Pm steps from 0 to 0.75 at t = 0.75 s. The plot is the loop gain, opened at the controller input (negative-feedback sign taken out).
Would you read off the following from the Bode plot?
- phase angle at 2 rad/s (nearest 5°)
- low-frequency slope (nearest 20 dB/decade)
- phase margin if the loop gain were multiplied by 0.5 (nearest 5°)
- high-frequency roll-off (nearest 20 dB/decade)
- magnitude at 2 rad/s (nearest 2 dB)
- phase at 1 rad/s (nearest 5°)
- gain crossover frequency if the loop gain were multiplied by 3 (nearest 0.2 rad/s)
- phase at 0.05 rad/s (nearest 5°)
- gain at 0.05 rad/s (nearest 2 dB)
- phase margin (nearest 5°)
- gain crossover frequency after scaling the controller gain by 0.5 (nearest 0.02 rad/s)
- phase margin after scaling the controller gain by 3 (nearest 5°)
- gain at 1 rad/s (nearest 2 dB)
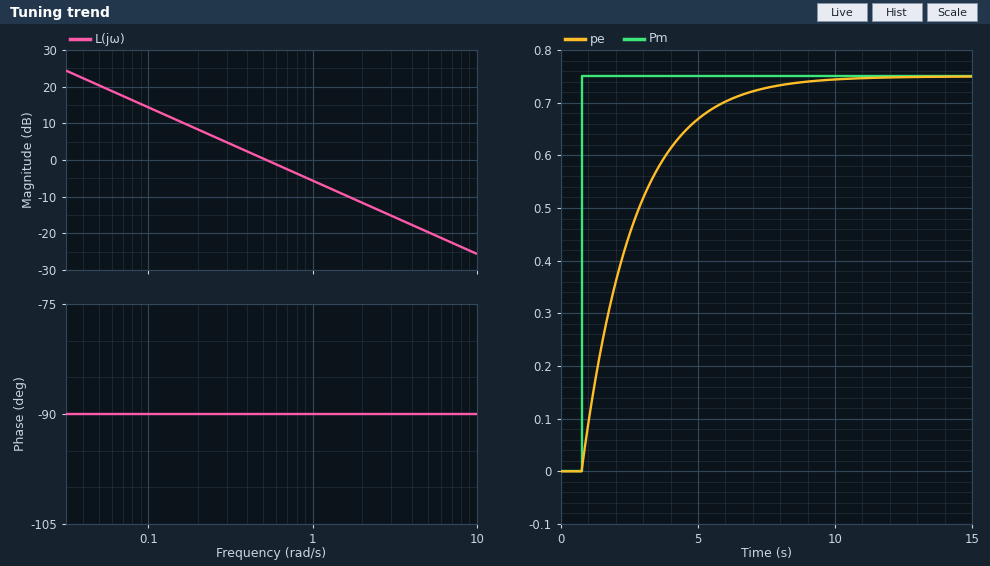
-90°
-20 dB/decade
90°
-20 dB/decade
-12 dB
-90°
1.6 rad/s
-90°
20 dB
90°
0.26 rad/s
90°
-6 dB
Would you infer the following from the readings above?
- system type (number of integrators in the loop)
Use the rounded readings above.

1
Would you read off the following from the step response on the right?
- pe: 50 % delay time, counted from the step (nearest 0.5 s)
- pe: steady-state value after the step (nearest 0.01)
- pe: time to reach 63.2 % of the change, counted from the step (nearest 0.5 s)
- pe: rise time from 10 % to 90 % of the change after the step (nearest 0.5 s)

1.5 s
0.75
2.0 s
4.0 s
